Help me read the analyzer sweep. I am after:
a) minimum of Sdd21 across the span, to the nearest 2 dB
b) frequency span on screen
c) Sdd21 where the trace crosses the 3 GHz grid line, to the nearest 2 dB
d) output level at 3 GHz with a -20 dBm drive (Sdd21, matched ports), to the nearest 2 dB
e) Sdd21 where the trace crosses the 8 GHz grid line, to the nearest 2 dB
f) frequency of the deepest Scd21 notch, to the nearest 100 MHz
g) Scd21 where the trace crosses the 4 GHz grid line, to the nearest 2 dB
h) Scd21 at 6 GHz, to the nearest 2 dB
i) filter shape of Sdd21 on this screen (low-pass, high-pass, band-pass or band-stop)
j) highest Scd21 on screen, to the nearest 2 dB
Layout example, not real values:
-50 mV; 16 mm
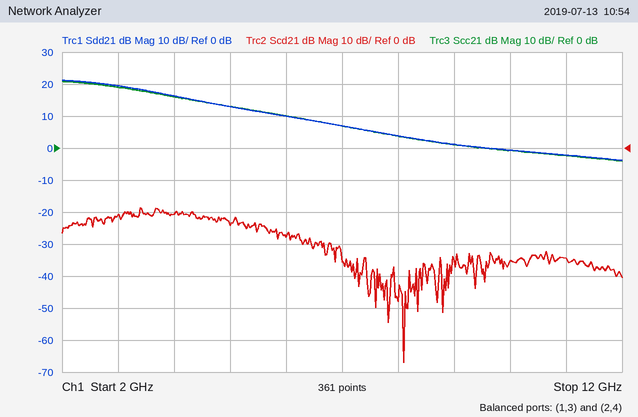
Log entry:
-4 dB; 10 GHz; 20 dB; 0 dBm; 4 dB; 8.1 GHz; -20 dB; -28 dB; low-pass; -18 dB
